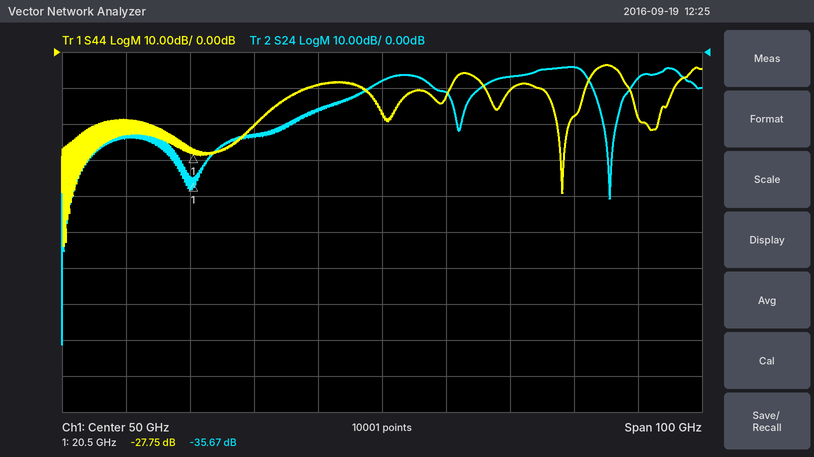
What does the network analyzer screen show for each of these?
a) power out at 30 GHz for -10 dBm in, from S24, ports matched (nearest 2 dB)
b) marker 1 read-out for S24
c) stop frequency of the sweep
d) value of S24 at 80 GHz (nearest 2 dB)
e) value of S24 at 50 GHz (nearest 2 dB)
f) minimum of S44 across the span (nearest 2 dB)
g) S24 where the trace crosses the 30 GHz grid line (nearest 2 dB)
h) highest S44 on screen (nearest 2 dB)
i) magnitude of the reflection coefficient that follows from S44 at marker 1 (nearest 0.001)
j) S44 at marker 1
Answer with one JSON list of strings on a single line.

["-34 dBm", "-35.67 dB", "100 GHz", "-4 dB", "-8 dB", "-54 dB", "-24 dB", "-4 dB", "0.041", "-27.75 dB"]
